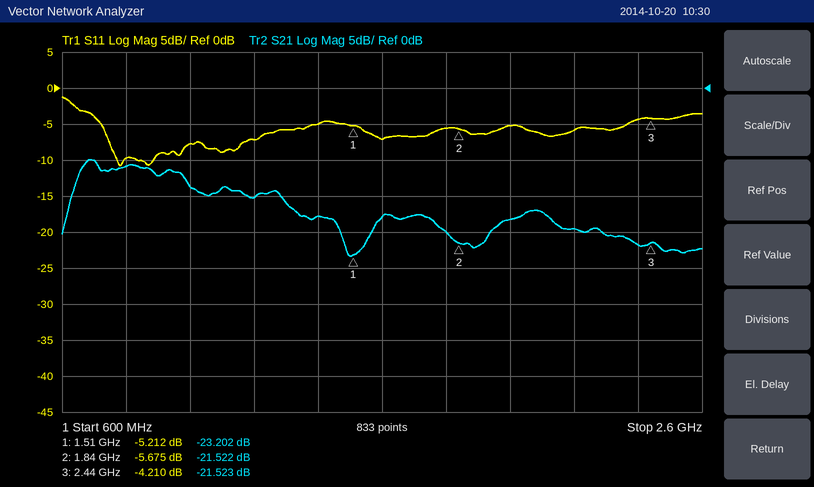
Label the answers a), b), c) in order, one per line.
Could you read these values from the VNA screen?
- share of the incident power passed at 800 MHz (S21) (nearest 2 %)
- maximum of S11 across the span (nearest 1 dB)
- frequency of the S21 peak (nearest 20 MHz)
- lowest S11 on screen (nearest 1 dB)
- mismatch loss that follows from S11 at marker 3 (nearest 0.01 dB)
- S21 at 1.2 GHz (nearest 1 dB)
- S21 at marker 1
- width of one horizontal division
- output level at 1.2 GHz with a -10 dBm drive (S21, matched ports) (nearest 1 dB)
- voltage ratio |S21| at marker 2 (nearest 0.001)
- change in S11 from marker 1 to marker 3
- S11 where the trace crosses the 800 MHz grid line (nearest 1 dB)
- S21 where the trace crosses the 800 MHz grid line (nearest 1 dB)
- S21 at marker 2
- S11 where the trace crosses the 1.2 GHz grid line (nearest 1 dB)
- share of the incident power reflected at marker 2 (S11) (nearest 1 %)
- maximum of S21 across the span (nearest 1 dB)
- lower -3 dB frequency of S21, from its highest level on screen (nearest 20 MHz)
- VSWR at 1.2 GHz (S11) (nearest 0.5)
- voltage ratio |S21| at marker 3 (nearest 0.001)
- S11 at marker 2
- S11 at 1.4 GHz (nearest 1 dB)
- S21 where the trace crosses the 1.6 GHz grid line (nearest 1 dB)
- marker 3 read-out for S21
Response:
a) 8 %
b) -1 dB
c) 680 MHz
d) -11 dB
e) 2.07 dB
f) -15 dB
g) -23.202 dB
h) 200 MHz
i) -25 dBm
j) 0.084
k) 1.002 dB
l) -10 dB
m) -11 dB
n) -21.522 dB
o) -7 dB
p) 27 %
q) -10 dB
r) 640 MHz
s) 2.5
t) 0.084
u) -5.675 dB
v) -5 dB
w) -18 dB
x) -21.523 dB
